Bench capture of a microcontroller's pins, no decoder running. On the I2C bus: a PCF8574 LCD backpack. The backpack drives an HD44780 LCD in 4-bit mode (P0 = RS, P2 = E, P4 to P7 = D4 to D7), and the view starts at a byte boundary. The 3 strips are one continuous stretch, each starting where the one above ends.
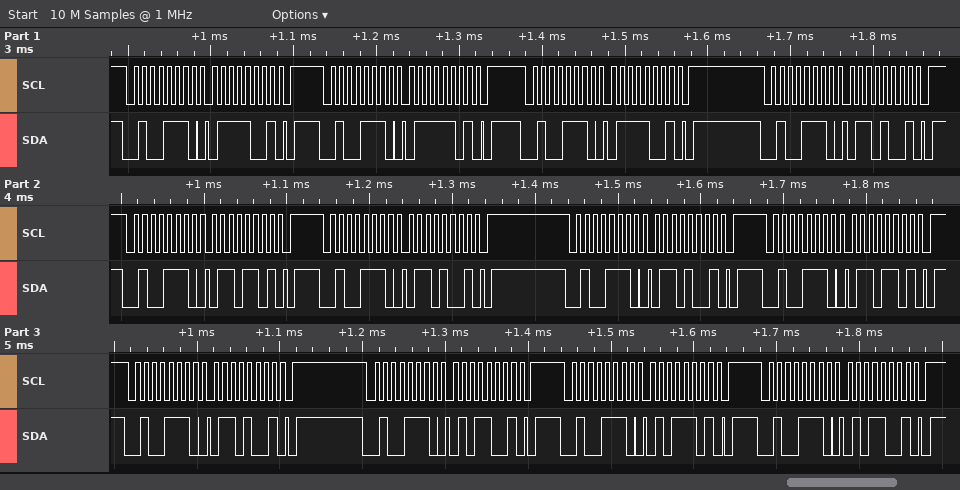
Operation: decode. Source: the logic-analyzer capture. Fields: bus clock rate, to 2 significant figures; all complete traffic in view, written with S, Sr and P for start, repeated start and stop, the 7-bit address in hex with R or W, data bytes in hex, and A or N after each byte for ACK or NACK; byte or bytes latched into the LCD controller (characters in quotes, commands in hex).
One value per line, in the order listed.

100 kHz
S 27W A 79 A P S 27W A 7D A P S 27W A 79 A P S 27W A 69 A P S 27W A 6D A P S 27W A 69 A P S 27W A 69 A P S 27W A 6D A P S 27W A 69 A P S 27W A 59 A P S 27W A 5D A P S 27W A 59 A P
'v' 'e'
